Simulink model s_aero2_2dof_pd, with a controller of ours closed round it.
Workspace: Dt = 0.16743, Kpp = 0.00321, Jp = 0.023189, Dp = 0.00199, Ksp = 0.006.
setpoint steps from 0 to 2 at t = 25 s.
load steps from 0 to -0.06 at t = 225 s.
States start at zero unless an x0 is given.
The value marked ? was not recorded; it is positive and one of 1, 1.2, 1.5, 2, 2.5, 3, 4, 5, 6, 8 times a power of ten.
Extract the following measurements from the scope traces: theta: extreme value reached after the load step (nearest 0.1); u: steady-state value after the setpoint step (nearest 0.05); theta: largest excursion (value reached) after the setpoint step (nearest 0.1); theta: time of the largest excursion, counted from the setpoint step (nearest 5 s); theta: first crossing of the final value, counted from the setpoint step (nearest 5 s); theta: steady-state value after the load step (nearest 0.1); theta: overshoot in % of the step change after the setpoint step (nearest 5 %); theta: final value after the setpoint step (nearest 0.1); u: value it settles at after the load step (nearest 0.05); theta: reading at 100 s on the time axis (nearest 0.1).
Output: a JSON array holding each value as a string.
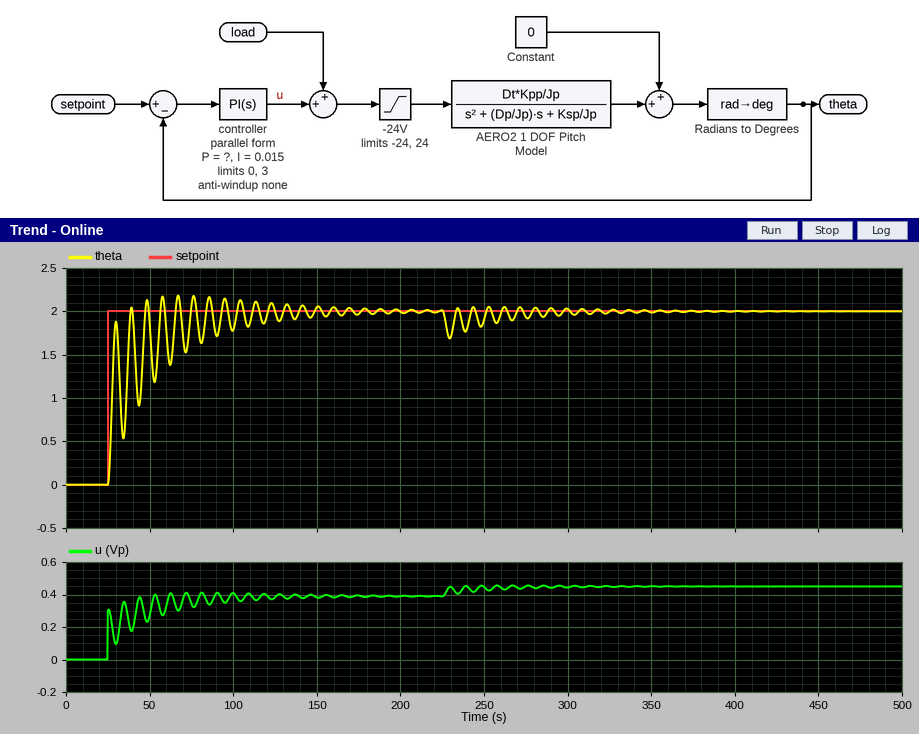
["1.7", "0.40", "2.2", "40 s", "15 s", "2.0", "10 %", "2.0", "0.45", "1.8"]
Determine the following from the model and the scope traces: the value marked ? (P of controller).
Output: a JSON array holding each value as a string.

["0.15"]
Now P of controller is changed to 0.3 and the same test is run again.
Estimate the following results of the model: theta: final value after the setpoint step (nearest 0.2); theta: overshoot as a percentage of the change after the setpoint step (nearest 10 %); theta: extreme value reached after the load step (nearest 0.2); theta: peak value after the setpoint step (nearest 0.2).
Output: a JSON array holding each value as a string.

["2.0", "20 %", "1.8", "2.4"]
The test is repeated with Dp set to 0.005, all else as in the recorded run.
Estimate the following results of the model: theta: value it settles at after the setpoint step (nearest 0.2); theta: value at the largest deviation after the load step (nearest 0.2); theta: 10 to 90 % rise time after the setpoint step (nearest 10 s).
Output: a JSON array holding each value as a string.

["2.0", "1.8", "40 s"]
